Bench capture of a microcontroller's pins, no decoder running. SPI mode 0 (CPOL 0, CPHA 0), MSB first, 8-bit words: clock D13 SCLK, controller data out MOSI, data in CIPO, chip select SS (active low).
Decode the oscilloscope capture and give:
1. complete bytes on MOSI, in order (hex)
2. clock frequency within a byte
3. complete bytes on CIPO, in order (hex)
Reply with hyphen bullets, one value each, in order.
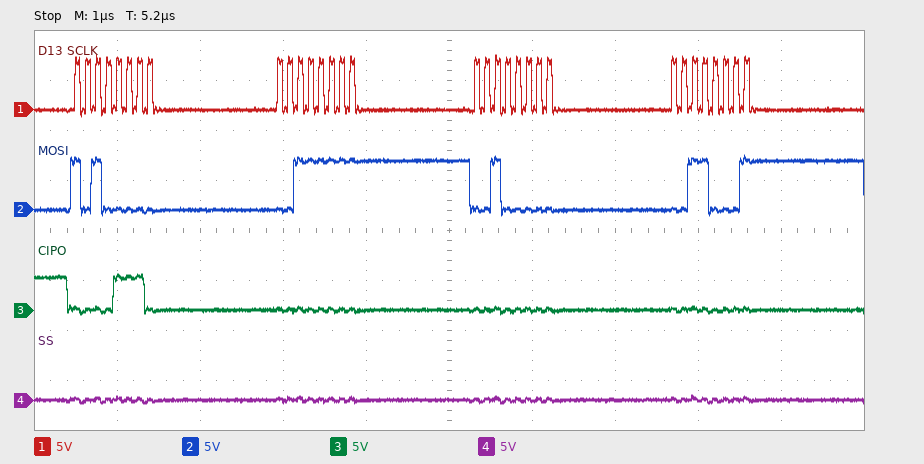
- A0 3F 20 31
- 8 MHz
- 0E 00 00 00
